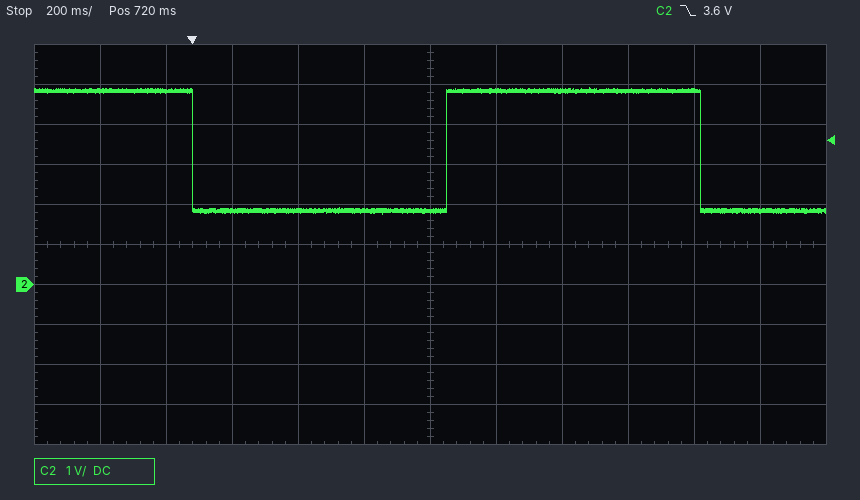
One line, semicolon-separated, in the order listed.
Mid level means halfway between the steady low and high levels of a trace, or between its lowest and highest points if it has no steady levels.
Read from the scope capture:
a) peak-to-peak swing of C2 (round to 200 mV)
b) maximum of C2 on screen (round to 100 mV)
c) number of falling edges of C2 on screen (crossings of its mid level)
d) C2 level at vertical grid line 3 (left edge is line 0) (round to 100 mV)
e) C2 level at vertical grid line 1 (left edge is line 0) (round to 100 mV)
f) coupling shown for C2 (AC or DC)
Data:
3.2 V; 4.9 V; 2; 1.8 V; 4.8 V; DC
